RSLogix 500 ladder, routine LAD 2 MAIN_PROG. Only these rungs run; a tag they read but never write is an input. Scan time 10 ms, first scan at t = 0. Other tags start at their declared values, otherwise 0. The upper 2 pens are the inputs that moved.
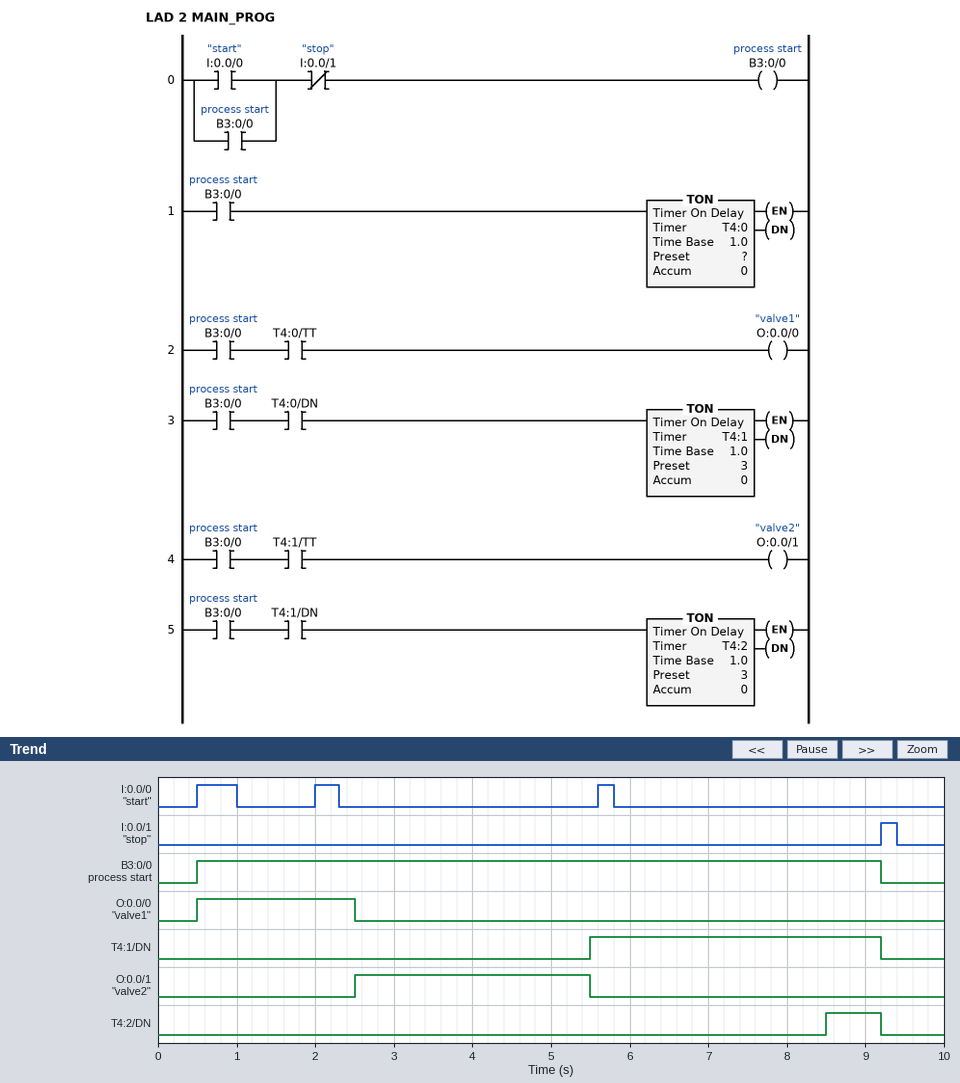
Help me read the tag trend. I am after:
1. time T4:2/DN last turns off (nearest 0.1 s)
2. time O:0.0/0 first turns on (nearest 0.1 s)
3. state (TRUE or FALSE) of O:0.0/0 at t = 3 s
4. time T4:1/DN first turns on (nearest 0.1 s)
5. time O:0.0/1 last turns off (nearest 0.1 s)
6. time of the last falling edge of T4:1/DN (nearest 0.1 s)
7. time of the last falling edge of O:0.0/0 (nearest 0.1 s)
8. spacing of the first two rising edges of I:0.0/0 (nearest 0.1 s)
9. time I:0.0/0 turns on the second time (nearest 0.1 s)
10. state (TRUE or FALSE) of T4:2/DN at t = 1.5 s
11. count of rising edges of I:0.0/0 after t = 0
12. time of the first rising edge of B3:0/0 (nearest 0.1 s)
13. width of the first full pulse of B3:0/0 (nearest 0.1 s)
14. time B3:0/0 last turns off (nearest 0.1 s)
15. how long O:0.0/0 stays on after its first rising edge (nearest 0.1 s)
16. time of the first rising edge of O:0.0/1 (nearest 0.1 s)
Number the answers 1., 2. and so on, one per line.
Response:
1. 9.2 s
2. 0.5 s
3. FALSE
4. 5.5 s
5. 5.5 s
6. 9.2 s
7. 2.5 s
8. 1.5 s
9. 2.0 s
10. FALSE
11. 3
12. 0.5 s
13. 8.7 s
14. 9.2 s
15. 2.0 s
16. 2.5 s
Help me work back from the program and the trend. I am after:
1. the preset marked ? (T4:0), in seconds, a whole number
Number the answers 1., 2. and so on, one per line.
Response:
1. 2 s
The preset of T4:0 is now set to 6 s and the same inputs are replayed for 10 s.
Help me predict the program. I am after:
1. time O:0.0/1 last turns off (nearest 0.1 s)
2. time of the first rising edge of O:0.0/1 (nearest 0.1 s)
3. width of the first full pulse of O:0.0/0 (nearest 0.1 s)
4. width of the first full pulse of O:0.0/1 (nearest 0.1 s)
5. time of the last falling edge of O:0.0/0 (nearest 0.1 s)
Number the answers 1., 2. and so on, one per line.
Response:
1. 9.2 s
2. 6.5 s
3. 6.0 s
4. 2.7 s
5. 6.5 s
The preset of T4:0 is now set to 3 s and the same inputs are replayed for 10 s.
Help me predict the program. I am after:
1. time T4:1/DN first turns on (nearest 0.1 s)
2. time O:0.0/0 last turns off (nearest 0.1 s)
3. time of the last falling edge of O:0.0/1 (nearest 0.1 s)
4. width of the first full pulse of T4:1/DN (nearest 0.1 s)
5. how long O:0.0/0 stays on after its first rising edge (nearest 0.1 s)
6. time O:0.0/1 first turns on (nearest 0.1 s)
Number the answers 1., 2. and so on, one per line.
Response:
1. 6.5 s
2. 3.5 s
3. 6.5 s
4. 2.7 s
5. 3.0 s
6. 3.5 s
